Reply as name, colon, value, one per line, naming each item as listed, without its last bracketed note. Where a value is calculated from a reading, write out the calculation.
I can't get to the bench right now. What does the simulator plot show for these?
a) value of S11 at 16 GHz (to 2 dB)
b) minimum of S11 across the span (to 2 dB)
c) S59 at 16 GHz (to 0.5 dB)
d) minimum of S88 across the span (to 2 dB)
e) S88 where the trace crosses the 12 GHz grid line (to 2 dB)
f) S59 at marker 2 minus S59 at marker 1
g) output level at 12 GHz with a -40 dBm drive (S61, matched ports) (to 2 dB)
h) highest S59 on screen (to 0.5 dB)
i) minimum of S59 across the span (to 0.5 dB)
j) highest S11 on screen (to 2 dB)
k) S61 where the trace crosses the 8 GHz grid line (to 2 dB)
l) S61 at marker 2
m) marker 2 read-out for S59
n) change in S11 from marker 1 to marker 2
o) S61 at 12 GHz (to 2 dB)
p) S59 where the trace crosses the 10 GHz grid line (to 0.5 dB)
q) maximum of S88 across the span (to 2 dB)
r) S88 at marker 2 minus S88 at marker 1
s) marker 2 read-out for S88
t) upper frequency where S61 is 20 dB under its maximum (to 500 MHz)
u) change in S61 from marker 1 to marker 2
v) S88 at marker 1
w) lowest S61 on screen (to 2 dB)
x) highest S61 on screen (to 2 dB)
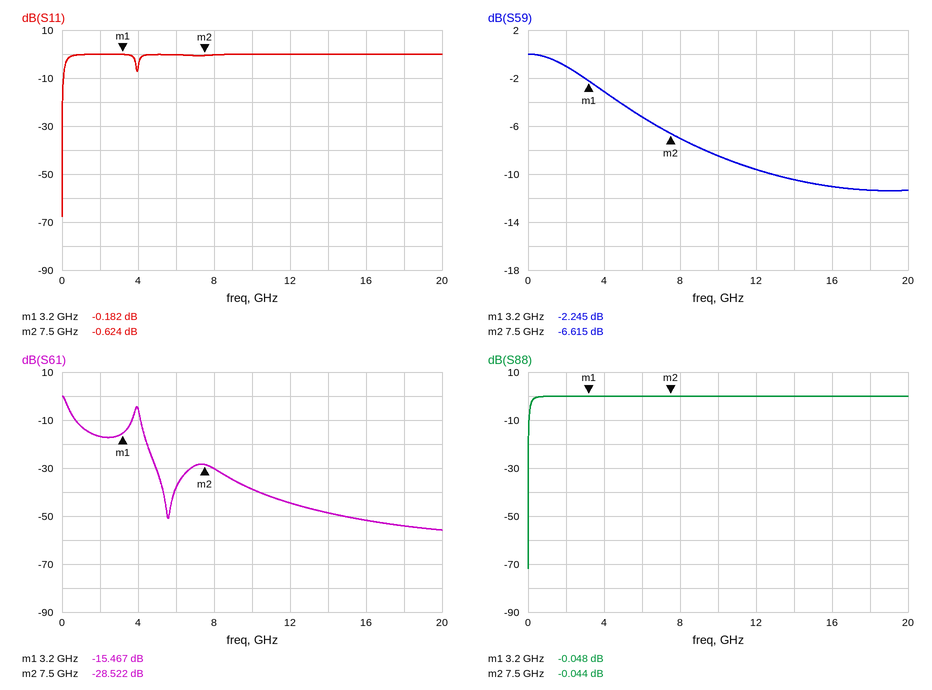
value of S11 at 16 GHz: 0 dB
minimum of S11 across the span: -68 dB
S59 at 16 GHz: -11.0 dB
minimum of S88 across the span: -72 dB
S88 where the trace crosses the 12 GHz grid line: 0 dB
S59 at marker 2 minus S59 at marker 1: -6.615 − (-2.245) = -4.370 dB
output level at 12 GHz with a -40 dBm drive (S61, matched ports): -40 dBm + (-44 dB) = -84 dBm
highest S59 on screen: 0.0 dB
minimum of S59 across the span: -11.5 dB
highest S11 on screen: 0 dB
S61 where the trace crosses the 8 GHz grid line: -30 dB
S61 at marker 2: -28.522 dB
marker 2 read-out for S59: -6.615 dB
change in S11 from marker 1 to marker 2: -0.624 − (-0.182) = -0.442 dB
S61 at 12 GHz: -44 dB
S59 where the trace crosses the 10 GHz grid line: -8.5 dB
maximum of S88 across the span: 0 dB
S88 at marker 2 minus S88 at marker 1: -0.044 − (-0.048) = 0.004 dB
marker 2 read-out for S88: -0.044 dB
upper frequency where S61 is 20 dB under its maximum: 4.5 GHz
change in S61 from marker 1 to marker 2: -28.522 − (-15.467) = -13.055 dB
S88 at marker 1: -0.048 dB
lowest S61 on screen: -56 dB
highest S61 on screen: 0 dB
